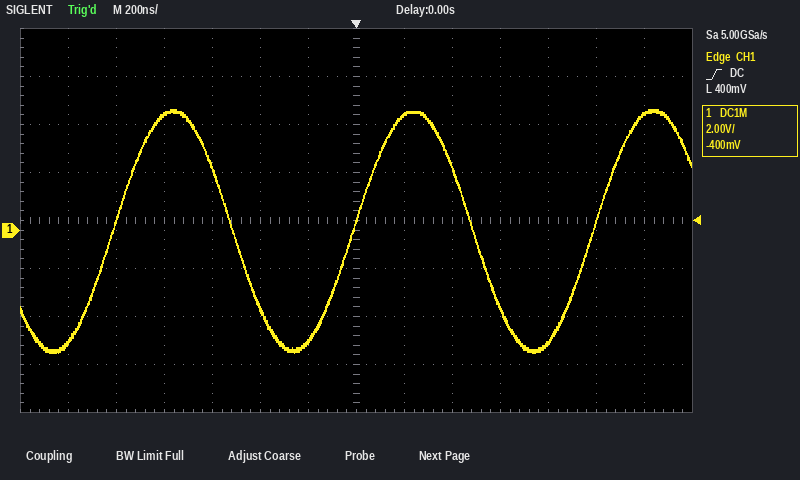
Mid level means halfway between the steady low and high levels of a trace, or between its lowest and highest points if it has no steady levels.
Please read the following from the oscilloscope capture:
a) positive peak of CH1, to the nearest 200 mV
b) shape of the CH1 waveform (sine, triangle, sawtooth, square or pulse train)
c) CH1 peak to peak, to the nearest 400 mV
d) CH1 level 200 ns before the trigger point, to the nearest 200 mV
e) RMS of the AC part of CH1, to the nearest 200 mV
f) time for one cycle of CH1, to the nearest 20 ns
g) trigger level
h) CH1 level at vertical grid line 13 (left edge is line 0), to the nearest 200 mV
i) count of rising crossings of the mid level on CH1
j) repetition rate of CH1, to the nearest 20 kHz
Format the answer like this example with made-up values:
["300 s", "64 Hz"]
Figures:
["5.0 V", "sine", "10.0 V", "-4.6 V", "3.6 V", "1.00 µs", "400 mV", "4.8 V", "3", "1.00 MHz"]
